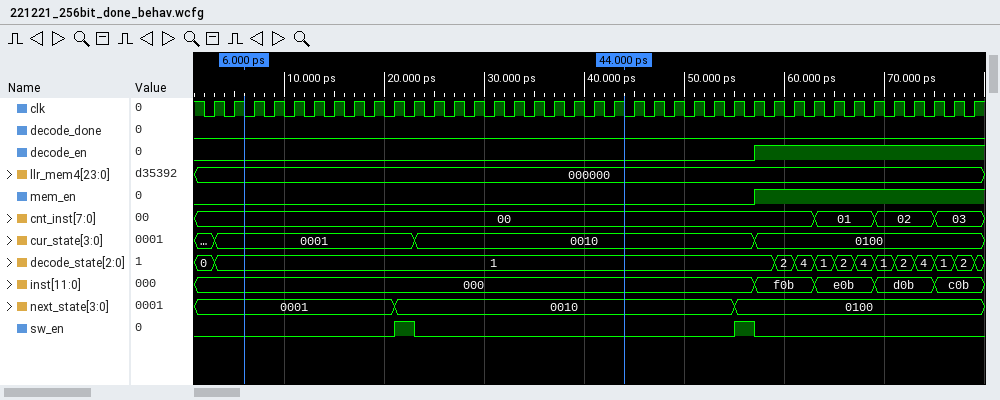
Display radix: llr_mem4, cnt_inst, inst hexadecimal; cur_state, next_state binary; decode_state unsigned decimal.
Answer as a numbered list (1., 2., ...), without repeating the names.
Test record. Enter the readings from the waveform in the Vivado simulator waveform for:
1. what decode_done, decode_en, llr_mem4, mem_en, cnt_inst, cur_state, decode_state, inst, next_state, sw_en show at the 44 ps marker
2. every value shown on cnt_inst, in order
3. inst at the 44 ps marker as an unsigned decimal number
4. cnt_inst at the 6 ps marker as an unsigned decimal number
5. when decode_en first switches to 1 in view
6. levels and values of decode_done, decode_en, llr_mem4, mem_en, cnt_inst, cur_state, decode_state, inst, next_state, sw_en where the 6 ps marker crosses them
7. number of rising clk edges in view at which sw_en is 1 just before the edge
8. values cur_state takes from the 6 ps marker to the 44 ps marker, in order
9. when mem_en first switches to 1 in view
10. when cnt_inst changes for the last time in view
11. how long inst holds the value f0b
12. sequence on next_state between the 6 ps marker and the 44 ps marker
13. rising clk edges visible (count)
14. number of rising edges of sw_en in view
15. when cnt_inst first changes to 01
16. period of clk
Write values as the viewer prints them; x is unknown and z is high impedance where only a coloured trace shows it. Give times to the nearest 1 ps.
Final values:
1. decode_done=0, decode_en=0, llr_mem4=000000, mem_en=0, cnt_inst=00, cur_state=0010, decode_state=1, inst=000, next_state=0010, sw_en=0
2. 00, 01, 02, 03
3. 0
4. 0
5. 57 ps
6. decode_done=0, decode_en=0, llr_mem4=000000, mem_en=0, cnt_inst=00, cur_state=0001, decode_state=1, inst=000, next_state=0001, sw_en=0
7. 2
8. 0001, 0010
9. 57 ps
10. 75 ps
11. 6 ps
12. 0001, 0010
13. 39
14. 2
15. 63 ps
16. 2 ps
